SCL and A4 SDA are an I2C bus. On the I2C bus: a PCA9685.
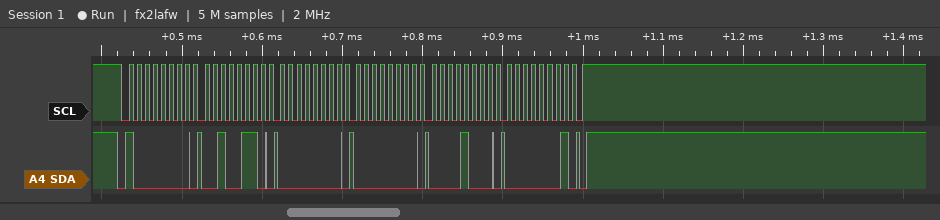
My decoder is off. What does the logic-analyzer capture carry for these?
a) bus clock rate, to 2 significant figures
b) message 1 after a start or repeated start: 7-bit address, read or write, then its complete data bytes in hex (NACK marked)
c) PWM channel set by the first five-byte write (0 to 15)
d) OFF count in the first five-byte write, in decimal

100 kHz
0x40 write: 26 00 00 08 01
8
264
